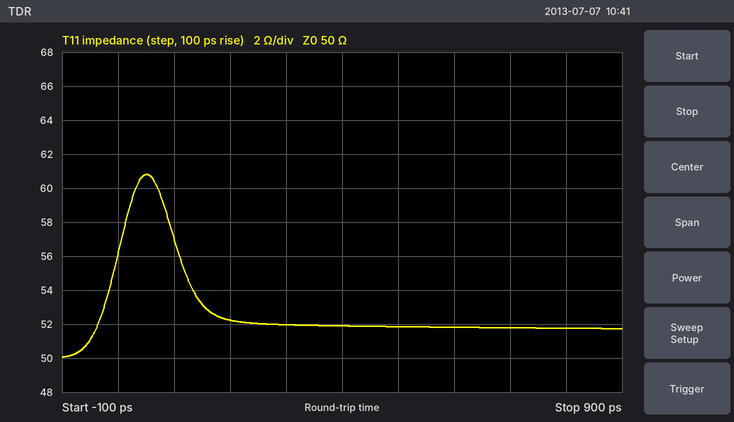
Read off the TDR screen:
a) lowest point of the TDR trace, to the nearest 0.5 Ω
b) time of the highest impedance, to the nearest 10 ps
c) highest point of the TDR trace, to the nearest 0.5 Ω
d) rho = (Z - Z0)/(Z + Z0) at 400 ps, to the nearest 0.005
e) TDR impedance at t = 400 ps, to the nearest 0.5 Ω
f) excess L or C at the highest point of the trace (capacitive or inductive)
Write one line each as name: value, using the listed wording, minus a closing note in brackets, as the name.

lowest point of the TDR trace, to the nearest 0.5 Ω: 50.0 Ω
time of the highest impedance, to the nearest 10 ps: 50 ps
highest point of the TDR trace, to the nearest 0.5 Ω: 61.0 Ω
rho = (Z - Z0)/(Z + Z0) at 400 ps, to the nearest 0.005: +0.020
TDR impedance at t = 400 ps, to the nearest 0.5 Ω: 52.0 Ω
excess L or C at the highest point of the trace: inductive
